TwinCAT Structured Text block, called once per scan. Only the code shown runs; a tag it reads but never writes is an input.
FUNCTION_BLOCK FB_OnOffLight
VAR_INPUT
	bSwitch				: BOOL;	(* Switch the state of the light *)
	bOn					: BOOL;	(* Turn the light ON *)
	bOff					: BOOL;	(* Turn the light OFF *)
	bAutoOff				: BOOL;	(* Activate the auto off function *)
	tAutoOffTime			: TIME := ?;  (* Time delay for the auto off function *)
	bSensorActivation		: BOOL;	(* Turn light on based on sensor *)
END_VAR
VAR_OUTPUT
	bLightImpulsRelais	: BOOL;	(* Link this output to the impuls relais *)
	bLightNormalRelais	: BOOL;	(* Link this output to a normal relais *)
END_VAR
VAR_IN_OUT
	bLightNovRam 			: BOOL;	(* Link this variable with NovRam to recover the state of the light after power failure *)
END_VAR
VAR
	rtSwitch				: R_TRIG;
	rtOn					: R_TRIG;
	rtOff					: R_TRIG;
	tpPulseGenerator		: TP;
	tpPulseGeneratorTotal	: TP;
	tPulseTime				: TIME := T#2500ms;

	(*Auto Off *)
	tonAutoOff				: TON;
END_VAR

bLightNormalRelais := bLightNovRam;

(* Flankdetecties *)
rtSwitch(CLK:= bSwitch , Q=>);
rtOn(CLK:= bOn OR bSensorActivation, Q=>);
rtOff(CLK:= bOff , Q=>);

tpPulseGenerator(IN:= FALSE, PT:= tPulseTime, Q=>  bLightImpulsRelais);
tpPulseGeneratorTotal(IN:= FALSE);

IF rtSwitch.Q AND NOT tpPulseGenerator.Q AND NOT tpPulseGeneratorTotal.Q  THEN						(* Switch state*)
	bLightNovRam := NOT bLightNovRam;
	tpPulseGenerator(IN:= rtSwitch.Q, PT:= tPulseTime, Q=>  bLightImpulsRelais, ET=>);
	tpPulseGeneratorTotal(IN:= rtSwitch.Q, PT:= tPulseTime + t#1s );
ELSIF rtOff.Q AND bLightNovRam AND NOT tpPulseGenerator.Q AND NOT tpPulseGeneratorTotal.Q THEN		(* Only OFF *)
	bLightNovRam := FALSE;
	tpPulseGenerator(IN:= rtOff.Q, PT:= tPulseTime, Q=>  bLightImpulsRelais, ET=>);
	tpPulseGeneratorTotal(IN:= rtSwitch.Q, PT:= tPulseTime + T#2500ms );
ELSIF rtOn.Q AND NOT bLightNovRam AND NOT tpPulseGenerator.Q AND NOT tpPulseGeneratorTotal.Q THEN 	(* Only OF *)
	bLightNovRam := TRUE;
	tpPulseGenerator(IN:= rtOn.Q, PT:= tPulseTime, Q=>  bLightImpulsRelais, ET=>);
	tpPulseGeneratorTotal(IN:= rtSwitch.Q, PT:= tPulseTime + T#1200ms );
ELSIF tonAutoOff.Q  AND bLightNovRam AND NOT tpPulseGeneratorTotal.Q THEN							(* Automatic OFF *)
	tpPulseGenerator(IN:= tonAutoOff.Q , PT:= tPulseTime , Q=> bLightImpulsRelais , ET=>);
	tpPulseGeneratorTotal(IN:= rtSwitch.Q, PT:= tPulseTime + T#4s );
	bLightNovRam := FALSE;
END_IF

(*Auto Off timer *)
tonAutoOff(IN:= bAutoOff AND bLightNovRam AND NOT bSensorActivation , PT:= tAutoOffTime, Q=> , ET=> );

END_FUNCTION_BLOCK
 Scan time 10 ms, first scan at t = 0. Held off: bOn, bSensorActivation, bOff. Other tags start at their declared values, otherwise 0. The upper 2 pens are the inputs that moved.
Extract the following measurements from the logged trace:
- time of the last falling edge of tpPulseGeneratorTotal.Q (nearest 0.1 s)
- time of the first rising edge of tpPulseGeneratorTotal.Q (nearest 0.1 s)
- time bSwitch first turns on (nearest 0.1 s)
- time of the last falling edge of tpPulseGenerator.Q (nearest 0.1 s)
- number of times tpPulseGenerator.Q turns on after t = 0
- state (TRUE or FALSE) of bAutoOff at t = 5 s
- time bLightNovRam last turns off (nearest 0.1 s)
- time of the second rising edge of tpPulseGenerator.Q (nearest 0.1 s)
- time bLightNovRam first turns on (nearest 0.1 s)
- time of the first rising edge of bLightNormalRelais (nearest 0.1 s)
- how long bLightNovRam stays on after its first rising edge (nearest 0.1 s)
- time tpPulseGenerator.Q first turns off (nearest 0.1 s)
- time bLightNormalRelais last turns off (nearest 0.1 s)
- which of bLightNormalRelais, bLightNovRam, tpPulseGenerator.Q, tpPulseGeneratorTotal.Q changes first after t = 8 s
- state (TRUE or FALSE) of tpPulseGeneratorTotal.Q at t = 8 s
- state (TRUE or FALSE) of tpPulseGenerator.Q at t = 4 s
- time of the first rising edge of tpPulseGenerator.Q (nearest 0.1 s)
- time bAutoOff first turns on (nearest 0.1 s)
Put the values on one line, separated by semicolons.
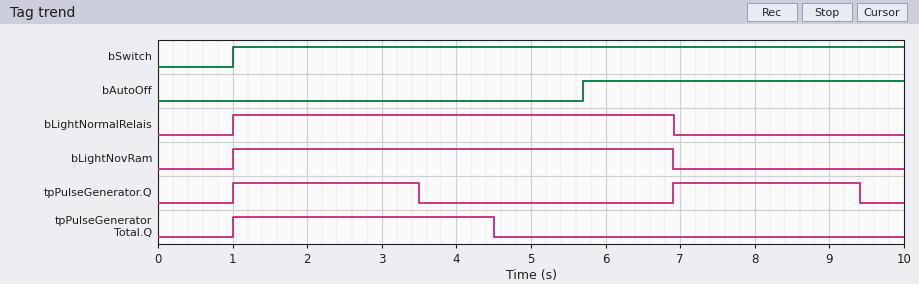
4.5 s; 1.0 s; 1.0 s; 9.4 s; 2; FALSE; 6.9 s; 6.9 s; 1.0 s; 1.0 s; 5.9 s; 3.5 s; 6.9 s; tpPulseGenerator.Q; FALSE; FALSE; 1.0 s; 5.7 s
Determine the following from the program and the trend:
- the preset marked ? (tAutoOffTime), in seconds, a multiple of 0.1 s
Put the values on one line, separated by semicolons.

1.2 s
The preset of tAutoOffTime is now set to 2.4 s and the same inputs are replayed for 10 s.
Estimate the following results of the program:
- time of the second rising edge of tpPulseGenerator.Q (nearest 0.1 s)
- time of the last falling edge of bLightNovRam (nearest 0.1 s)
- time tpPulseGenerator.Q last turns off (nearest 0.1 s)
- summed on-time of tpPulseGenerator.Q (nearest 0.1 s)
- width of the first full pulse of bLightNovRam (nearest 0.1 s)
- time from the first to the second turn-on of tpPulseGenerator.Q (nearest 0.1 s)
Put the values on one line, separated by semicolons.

8.1 s; 8.1 s; 3.5 s; 4.4 s; 7.1 s; 7.1 s
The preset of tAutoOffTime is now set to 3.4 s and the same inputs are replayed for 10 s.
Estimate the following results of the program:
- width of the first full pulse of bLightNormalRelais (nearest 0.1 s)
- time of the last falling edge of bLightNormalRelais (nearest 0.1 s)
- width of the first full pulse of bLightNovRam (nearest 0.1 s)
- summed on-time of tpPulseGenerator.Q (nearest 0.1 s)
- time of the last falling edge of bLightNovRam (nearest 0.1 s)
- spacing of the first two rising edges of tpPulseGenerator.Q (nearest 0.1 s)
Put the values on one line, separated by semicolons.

8.1 s; 9.1 s; 8.1 s; 3.4 s; 9.1 s; 8.1 s
